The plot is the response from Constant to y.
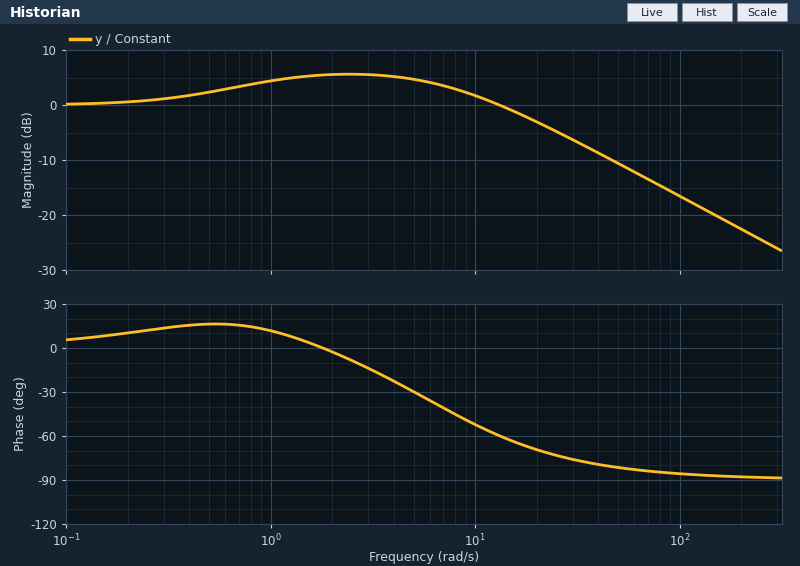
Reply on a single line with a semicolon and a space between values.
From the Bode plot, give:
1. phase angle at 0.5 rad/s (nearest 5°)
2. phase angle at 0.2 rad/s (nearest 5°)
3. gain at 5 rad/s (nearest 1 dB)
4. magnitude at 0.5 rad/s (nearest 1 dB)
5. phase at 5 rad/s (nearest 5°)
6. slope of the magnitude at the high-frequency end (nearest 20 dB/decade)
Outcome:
15°; 10°; 5 dB; 2 dB; -30°; -20 dB/decade
